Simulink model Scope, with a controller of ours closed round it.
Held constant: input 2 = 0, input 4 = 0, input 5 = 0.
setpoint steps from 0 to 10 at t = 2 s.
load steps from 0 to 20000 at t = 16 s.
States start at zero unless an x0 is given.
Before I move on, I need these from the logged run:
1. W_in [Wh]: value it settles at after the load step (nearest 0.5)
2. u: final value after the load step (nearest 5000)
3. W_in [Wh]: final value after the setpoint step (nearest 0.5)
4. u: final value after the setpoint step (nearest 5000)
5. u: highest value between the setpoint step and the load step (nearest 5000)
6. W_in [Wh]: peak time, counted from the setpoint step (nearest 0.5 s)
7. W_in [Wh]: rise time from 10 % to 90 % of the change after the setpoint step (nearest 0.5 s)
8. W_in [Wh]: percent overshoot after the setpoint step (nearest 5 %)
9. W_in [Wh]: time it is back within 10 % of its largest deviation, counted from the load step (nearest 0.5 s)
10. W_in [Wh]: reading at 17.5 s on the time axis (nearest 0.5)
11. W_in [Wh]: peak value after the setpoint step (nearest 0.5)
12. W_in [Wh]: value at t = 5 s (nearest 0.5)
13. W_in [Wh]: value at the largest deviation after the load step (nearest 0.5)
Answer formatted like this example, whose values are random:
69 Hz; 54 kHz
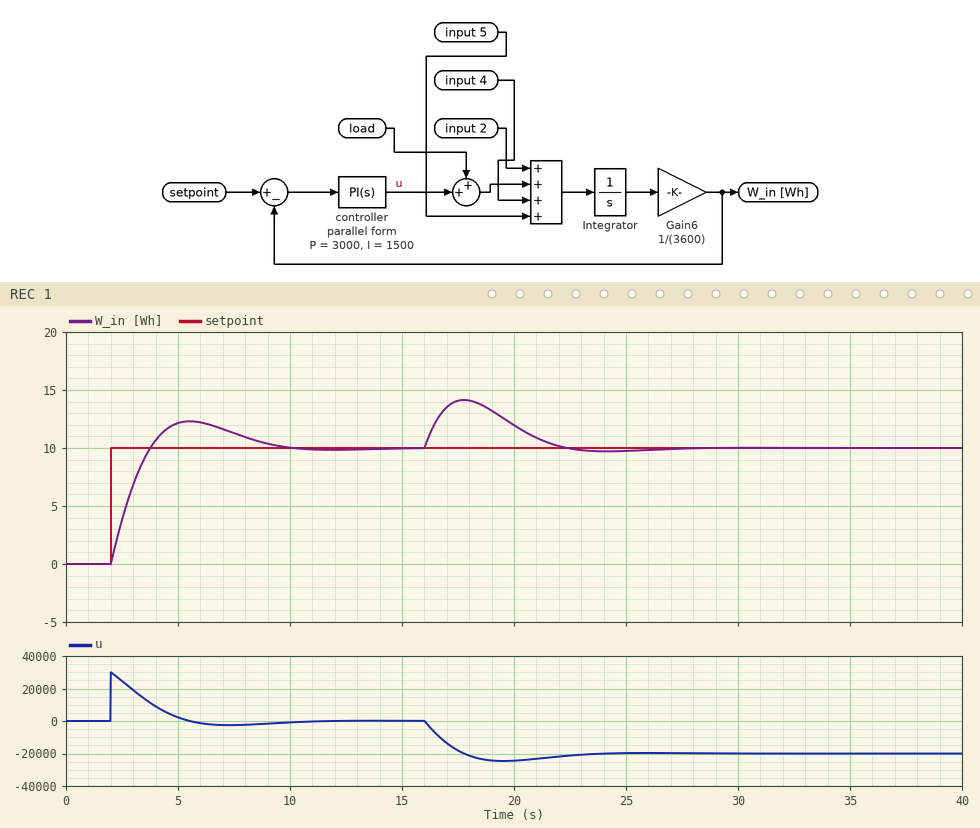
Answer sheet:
10.0; -20000; 10.0; 0; 30000; 3.5 s; 1.5 s; 25 %; 5.5 s; 14.0; 12.5; 12.0; 14.0
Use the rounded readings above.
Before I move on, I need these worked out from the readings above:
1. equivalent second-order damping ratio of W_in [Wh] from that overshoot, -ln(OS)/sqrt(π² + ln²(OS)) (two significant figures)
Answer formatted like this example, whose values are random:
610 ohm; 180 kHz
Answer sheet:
0.40
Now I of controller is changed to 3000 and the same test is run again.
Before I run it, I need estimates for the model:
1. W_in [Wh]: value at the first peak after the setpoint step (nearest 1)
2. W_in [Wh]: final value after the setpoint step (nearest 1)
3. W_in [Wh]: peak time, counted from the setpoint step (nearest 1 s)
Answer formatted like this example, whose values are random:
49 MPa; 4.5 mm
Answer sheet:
13; 10; 3 s
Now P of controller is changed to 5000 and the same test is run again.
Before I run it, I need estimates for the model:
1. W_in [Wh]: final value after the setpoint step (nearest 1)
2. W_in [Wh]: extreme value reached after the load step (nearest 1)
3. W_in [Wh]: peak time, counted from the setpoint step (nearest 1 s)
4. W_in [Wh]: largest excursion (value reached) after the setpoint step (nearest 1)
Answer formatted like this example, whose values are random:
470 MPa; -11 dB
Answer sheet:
10; 13; 3 s; 11
